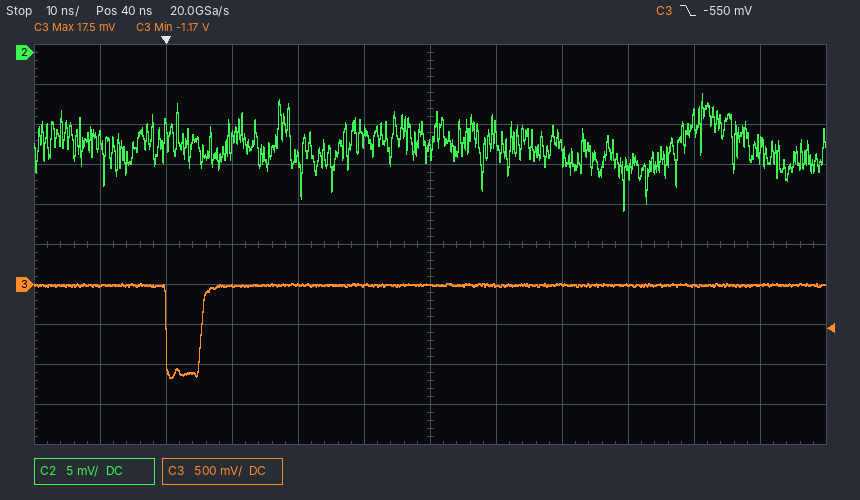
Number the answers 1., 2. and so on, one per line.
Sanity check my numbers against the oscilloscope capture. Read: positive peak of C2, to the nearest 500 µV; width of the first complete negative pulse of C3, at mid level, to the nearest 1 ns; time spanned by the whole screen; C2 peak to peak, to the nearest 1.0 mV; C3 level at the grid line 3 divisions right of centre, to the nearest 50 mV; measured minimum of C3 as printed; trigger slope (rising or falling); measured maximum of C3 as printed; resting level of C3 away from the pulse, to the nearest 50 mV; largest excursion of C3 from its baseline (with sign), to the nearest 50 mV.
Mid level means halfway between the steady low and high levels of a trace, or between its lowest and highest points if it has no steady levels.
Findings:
1. -5.0 mV
2. 5 ns
3. 120 ns
4. 15.0 mV
5. 0 mV
6. -1.17 V
7. falling
8. 17.5 mV
9. 0 mV
10. -1.15 V
